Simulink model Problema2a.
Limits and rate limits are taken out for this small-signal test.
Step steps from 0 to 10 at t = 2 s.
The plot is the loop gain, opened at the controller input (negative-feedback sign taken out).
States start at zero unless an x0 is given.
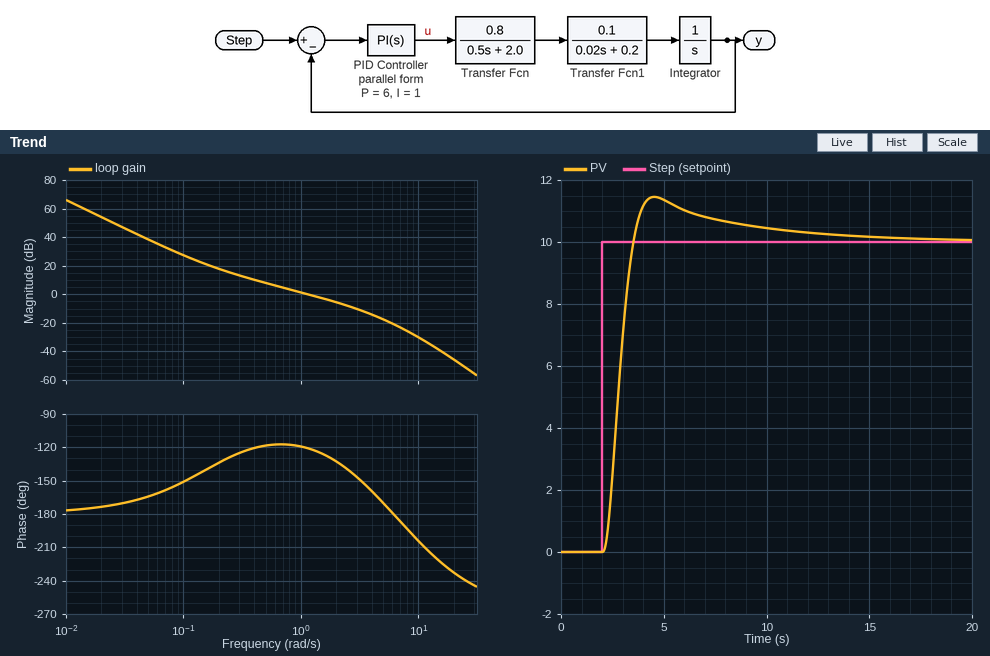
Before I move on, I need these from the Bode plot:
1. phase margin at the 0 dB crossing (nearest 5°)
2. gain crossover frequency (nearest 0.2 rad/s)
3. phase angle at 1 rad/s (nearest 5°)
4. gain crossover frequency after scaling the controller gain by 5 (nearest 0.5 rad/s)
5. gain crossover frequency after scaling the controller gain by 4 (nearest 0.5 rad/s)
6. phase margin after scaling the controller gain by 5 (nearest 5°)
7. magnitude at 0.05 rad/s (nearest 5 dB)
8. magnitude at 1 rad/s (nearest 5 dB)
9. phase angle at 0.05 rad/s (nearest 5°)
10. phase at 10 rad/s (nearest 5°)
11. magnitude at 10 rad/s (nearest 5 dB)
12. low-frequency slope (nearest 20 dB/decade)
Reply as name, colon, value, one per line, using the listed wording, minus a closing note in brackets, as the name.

phase margin at the 0 dB crossing: 60°
gain crossover frequency: 1.2 rad/s
phase angle at 1 rad/s: -120°
gain crossover frequency after scaling the controller gain by 5: 4.0 rad/s
gain crossover frequency after scaling the controller gain by 4: 3.5 rad/s
phase margin after scaling the controller gain by 5: 20°
magnitude at 0.05 rad/s: 40 dB
magnitude at 1 rad/s: 0 dB
phase angle at 0.05 rad/s: -165°
phase at 10 rad/s: -205°
magnitude at 10 rad/s: -30 dB
low-frequency slope: -40 dB/decade
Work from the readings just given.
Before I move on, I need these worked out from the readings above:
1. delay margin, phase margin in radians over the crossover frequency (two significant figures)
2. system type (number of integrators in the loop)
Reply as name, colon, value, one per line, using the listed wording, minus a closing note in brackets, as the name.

delay margin, phase margin in radians over the crossover frequency: 0.87 s
system type: 2
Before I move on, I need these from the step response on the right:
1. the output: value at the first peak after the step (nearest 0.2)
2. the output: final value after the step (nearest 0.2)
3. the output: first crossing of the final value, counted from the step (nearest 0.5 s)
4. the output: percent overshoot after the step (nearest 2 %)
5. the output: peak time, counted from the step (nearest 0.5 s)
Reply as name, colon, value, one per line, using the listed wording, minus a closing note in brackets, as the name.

the output: value at the first peak after the step: 11.4
the output: final value after the step: 10.0
the output: first crossing of the final value, counted from the step: 1.5 s
the output: percent overshoot after the step: 14 %
the output: peak time, counted from the step: 2.5 s
